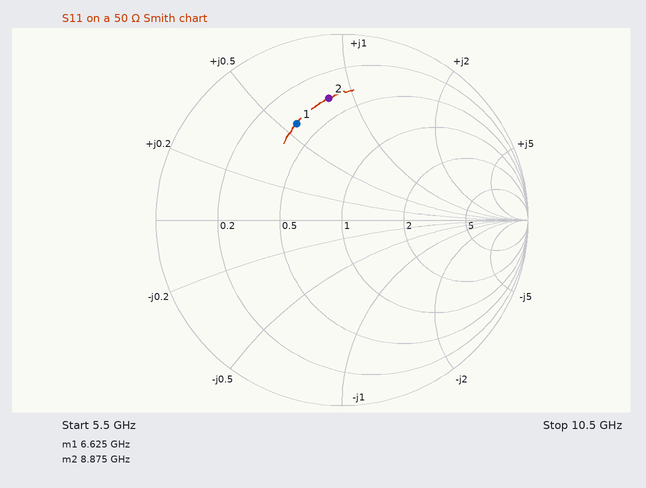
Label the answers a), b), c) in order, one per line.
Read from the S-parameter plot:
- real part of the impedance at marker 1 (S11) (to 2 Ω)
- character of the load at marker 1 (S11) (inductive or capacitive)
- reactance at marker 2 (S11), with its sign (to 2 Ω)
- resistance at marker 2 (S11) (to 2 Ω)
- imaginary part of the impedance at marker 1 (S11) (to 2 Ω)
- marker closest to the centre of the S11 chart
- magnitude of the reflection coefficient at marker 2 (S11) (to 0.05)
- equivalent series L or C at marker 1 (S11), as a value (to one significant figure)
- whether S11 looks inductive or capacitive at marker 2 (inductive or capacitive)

a) 18 Ω
b) inductive
c) +42 Ω
d) 18 Ω
e) +28 Ω
f) marker 1
g) 0.65
h) 700 pH
i) inductive
